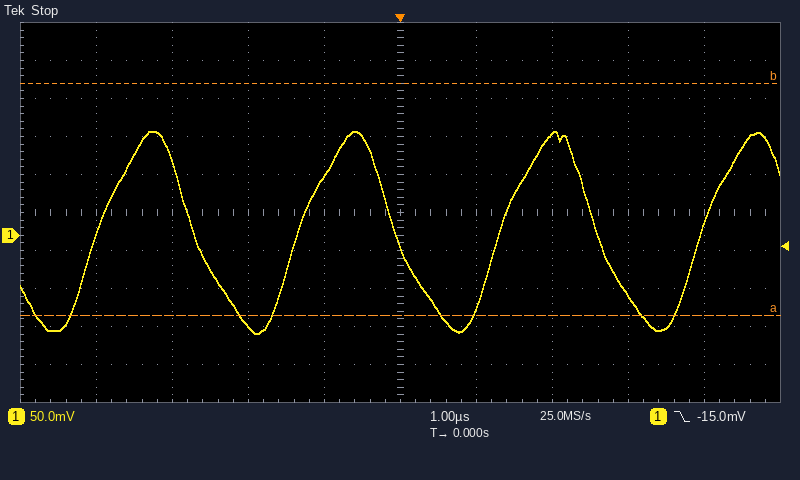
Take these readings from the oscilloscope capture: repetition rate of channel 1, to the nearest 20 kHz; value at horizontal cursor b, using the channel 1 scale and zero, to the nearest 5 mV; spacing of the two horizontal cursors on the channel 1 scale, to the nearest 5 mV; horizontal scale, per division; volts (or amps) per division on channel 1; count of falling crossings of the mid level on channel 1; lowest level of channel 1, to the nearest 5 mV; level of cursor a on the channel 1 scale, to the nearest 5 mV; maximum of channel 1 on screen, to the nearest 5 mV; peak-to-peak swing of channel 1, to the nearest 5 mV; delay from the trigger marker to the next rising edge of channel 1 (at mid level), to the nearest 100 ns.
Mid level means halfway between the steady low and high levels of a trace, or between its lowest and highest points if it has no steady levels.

380 kHz
200 mV
305 mV
1 µs
50 mV
3
-130 mV
-105 mV
135 mV
265 mV
1.3 µs
